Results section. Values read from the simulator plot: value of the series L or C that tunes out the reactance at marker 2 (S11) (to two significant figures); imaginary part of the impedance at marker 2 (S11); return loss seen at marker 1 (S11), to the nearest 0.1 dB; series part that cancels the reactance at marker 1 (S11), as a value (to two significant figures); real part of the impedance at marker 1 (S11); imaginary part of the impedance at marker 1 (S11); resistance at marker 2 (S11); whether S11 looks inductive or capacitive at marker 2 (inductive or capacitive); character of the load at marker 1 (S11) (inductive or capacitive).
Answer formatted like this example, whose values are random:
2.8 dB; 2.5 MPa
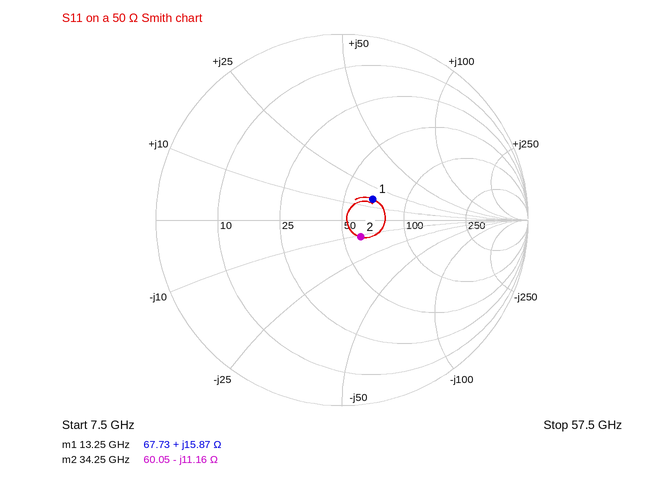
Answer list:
52 pH; -11.16 Ω; 14.0 dB; 760 fF; 67.73 Ω; +15.87 Ω; 60.05 Ω; capacitive; inductive
